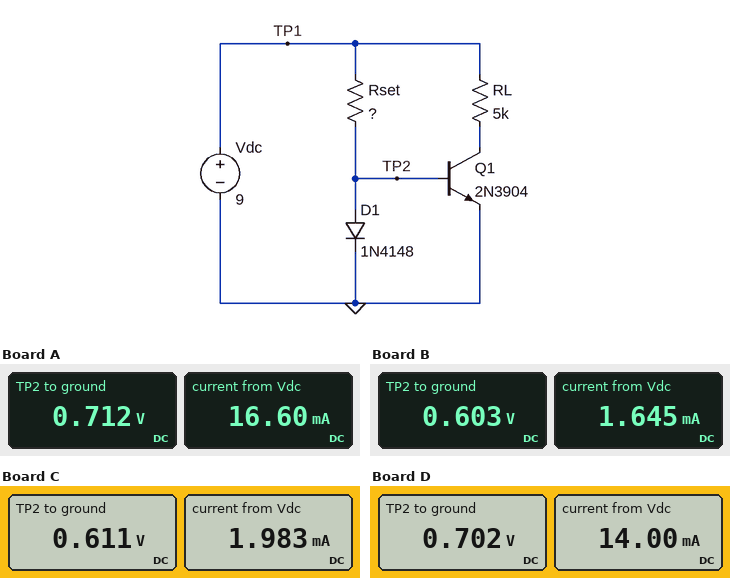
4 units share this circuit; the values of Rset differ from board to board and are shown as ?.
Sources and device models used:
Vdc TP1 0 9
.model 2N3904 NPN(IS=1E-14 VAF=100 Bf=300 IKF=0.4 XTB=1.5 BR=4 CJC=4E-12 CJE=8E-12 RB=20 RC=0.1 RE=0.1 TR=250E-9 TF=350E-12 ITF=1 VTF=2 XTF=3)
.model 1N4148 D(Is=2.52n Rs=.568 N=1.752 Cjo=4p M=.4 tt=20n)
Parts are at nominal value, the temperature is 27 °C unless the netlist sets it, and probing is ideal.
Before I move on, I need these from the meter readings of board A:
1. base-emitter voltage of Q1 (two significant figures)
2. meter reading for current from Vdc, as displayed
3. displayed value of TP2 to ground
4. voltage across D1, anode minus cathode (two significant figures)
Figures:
710 mV
16.60 mA
0.712 V
710 mV
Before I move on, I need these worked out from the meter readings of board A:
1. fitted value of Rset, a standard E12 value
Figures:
560 Ω
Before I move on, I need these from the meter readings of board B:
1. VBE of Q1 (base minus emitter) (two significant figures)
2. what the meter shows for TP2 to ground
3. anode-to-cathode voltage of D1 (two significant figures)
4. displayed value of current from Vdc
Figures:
600 mV
0.603 V
600 mV
1.645 mA
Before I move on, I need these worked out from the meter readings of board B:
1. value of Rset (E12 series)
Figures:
5.6 kΩ
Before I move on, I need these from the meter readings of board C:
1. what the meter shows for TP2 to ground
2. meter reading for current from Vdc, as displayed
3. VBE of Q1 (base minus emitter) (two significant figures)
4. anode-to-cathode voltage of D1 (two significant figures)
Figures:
0.611 V
1.983 mA
610 mV
610 mV
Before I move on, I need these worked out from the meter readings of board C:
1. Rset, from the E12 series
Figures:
4.7 kΩ
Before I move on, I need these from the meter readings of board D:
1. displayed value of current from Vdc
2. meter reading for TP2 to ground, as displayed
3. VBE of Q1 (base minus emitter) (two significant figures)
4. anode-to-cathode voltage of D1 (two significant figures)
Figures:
14.00 mA
0.702 V
700 mV
700 mV
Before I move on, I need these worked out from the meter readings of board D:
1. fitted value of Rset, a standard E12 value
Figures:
680 Ω
